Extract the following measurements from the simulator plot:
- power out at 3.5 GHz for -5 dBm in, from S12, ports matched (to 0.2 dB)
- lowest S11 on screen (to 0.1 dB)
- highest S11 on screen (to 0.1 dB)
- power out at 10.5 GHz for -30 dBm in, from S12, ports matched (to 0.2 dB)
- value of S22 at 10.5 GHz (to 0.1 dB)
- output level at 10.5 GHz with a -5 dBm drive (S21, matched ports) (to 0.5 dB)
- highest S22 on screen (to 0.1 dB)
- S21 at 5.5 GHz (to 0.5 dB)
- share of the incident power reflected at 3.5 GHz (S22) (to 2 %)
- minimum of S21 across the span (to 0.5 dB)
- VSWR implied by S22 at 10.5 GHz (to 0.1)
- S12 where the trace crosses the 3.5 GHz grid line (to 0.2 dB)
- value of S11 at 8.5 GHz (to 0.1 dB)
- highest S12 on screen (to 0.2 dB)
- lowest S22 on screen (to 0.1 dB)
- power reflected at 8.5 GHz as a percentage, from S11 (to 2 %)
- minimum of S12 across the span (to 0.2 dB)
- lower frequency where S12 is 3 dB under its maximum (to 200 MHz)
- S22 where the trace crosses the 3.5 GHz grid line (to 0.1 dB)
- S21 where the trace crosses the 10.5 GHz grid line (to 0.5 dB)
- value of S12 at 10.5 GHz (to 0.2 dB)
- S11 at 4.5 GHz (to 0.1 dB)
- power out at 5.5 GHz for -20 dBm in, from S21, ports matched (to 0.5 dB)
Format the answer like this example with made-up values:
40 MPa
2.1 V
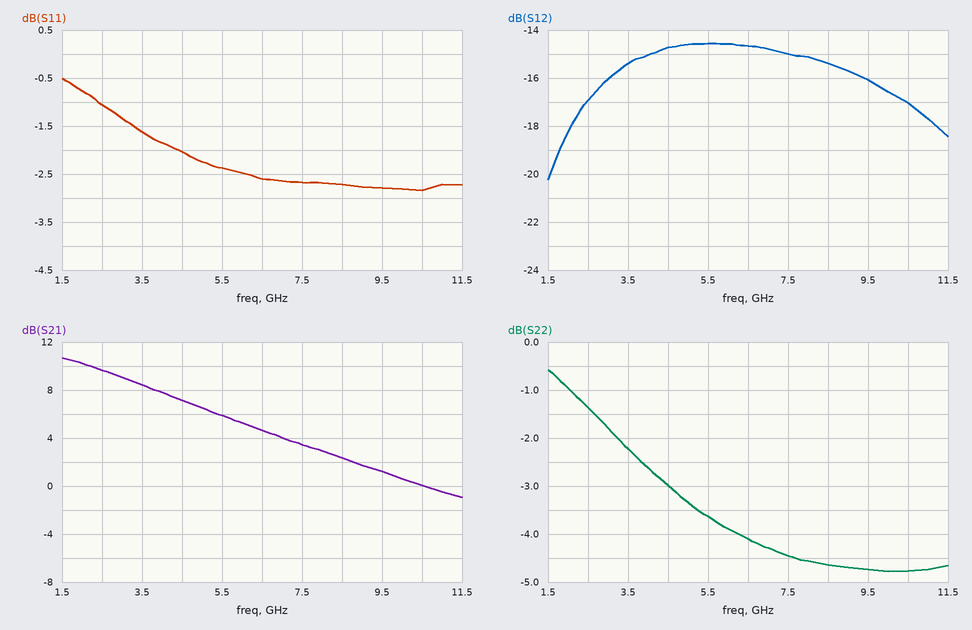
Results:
-20.4 dBm
-2.8 dB
-0.5 dB
-47.0 dBm
-4.8 dB
-5.0 dBm
-0.6 dB
6.0 dB
60 %
-1.0 dB
3.7
-15.4 dB
-2.7 dB
-14.6 dB
-4.8 dB
54 %
-20.2 dB
2.2 GHz
-2.2 dB
0.0 dB
-17.0 dB
-2.0 dB
-14.0 dBm
